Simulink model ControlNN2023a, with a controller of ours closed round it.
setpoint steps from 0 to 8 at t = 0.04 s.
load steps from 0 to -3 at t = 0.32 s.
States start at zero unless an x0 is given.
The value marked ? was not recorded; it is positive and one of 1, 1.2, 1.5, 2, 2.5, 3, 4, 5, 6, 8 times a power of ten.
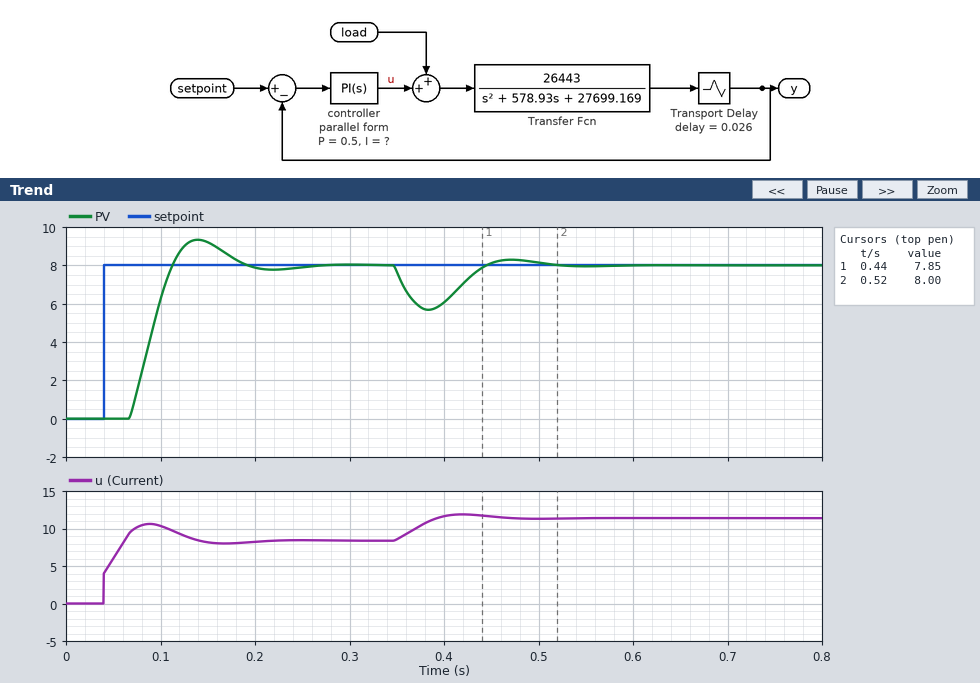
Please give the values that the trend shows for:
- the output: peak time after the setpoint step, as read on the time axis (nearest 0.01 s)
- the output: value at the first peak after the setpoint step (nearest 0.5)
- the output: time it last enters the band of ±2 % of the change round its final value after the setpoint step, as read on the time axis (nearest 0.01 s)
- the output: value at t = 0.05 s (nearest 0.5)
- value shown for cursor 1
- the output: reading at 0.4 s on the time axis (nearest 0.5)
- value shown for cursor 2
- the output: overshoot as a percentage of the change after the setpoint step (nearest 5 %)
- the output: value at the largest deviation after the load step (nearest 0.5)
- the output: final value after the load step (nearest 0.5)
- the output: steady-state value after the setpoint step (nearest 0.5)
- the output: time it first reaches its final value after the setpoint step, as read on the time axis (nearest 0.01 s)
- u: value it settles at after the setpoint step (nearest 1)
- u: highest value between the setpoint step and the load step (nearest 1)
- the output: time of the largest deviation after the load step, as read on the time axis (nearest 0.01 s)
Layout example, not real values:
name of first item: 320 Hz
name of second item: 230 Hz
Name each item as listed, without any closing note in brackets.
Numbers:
the output: peak time after the setpoint step, as read on the time axis: 0.14 s
the output: value at the first peak after the setpoint step: 9.5
the output: time it last enters the band of ±2 % of the change round its final value after the setpoint step, as read on the time axis: 0.24 s
the output: value at t = 0.05 s: 0.0
value shown for cursor 1: 7.85
the output: reading at 0.4 s on the time axis: 6.0
value shown for cursor 2: 8.00
the output: overshoot as a percentage of the change after the setpoint step: 15 %
the output: value at the largest deviation after the load step: 5.5
the output: final value after the load step: 8.0
the output: steady-state value after the setpoint step: 8.0
the output: time it first reaches its final value after the setpoint step, as read on the time axis: 0.11 s
u: value it settles at after the setpoint step: 8
u: highest value between the setpoint step and the load step: 11
the output: time of the largest deviation after the load step, as read on the time axis: 0.38 s
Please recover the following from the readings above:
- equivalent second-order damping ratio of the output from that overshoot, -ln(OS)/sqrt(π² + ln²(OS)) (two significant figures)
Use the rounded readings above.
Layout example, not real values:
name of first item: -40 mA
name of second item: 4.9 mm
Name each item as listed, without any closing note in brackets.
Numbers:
equivalent second-order damping ratio of the output from that overshoot, -ln(OS)/sqrt(π² + ln²(OS)): 0.52
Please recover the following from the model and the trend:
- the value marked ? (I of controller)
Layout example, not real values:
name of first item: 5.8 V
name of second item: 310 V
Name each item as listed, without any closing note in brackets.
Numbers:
the value marked ?: 25
